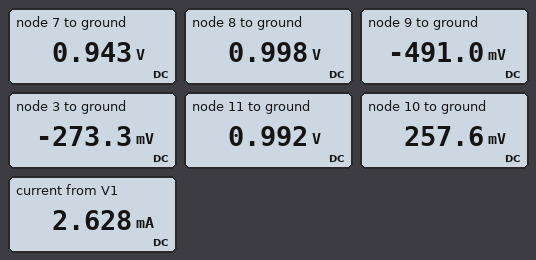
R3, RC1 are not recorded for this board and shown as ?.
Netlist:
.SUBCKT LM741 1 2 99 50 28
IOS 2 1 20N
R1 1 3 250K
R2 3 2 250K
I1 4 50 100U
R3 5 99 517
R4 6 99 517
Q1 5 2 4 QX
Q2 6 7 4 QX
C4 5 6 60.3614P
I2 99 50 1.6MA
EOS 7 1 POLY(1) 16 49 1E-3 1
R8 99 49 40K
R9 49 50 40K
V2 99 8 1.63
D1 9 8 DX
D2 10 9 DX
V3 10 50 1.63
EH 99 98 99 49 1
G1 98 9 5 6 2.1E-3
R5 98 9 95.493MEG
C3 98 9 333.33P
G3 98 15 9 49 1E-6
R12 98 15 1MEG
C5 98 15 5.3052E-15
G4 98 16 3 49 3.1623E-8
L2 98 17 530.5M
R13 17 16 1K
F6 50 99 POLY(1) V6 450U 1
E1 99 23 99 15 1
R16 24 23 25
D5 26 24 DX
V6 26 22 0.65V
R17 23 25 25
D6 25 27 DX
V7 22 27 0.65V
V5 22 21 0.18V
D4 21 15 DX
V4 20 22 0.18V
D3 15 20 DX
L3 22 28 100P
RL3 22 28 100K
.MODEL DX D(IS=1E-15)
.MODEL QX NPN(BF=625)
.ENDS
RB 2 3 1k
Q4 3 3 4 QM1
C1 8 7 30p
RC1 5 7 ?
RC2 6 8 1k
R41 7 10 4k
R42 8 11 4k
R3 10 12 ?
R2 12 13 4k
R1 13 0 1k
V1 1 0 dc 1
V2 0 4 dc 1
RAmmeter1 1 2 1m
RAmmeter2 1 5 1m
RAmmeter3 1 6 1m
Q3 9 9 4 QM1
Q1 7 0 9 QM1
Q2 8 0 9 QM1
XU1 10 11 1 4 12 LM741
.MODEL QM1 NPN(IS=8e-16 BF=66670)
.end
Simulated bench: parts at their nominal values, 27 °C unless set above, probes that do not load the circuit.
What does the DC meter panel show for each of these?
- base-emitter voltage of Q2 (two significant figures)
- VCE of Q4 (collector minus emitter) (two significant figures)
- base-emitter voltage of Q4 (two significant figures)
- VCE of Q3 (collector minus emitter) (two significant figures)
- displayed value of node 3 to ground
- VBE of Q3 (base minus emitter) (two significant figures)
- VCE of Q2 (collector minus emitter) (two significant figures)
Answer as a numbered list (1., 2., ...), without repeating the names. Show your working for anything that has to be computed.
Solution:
1. 0 V - (-491 mV) = 490 mV
2. -273.3 mV - (-1 V) = 730 mV
3. -273.3 mV - (-1 V) = 730 mV
4. -491 mV - (-1 V) = 510 mV
5. -273.3 mV
6. -491 mV - (-1 V) = 510 mV
7. 998 mV - (-491 mV) = 1.5 V
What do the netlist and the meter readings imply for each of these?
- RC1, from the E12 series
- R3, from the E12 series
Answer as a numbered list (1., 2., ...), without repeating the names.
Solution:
1. 330 Ω
2. 1.5 kΩ
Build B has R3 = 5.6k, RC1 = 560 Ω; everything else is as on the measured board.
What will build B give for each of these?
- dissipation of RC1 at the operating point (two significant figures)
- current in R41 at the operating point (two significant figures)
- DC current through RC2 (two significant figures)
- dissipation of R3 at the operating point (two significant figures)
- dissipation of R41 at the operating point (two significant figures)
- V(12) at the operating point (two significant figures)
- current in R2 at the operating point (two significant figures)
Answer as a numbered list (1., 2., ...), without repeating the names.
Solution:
1. 5.5 µW
2. 99 µA
3. 1.2 µA
4. 56 µW
5. 39 µW
6. -12 mV
7. 2.4 µA
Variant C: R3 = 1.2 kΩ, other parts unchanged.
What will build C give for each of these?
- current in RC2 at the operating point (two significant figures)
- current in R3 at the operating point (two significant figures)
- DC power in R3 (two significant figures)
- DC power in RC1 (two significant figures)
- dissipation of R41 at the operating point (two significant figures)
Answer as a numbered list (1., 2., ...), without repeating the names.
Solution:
1. 1.9 µA
2. 180 µA
3. 40 µW
4. 11 µW
5. 130 µW
